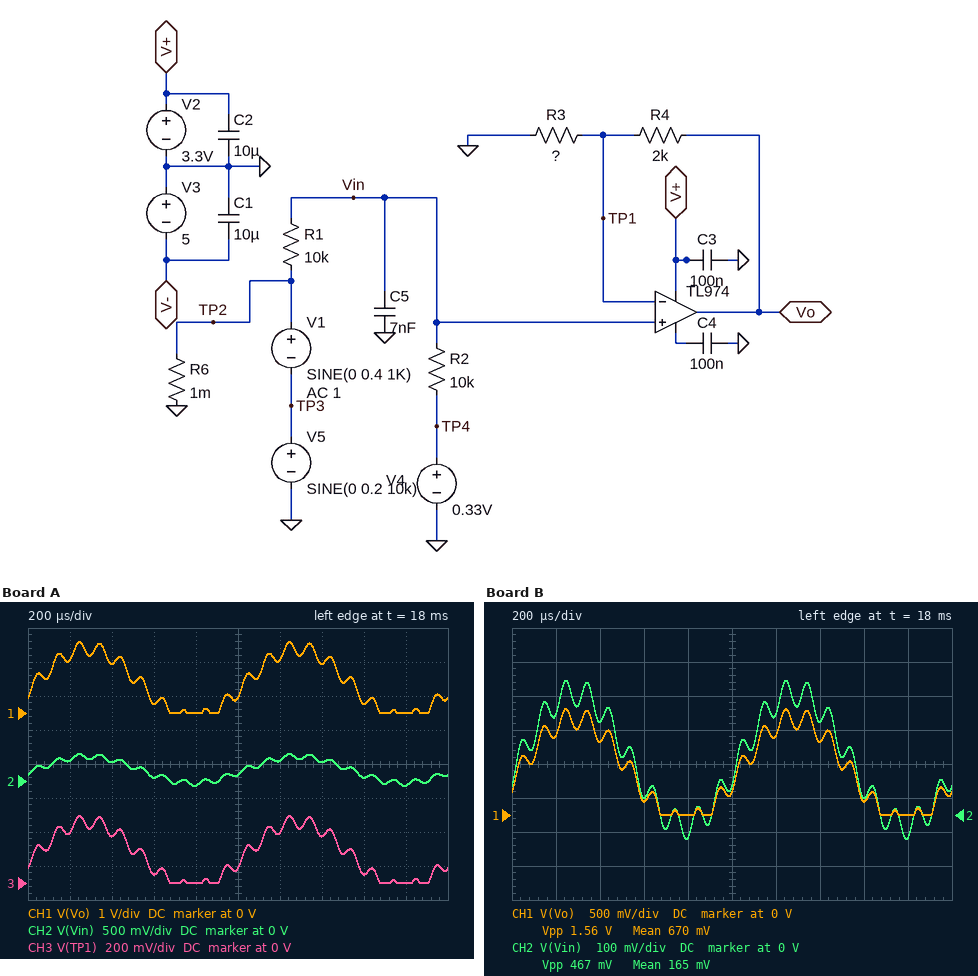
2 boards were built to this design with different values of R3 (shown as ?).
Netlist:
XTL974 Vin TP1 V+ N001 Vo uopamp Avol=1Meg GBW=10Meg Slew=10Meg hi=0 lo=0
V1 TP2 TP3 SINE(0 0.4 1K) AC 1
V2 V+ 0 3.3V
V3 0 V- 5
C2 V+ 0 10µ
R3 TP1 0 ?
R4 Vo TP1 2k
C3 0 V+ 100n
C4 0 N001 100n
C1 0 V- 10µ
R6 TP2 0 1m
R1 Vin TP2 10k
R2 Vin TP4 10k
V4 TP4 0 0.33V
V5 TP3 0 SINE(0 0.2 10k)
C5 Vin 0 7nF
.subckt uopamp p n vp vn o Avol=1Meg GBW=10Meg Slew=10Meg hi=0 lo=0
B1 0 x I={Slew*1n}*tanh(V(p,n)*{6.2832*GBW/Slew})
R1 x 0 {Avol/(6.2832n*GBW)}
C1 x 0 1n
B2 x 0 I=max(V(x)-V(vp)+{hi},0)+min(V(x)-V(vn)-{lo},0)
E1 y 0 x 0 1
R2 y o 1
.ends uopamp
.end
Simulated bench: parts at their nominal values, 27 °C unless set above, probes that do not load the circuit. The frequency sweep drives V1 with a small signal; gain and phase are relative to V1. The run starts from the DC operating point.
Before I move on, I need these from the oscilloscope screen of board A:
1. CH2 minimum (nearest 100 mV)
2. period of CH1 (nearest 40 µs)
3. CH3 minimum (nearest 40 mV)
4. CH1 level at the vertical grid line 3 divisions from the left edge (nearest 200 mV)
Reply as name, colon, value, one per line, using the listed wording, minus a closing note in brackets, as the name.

CH2 minimum: -100 mV
period of CH1: 1.00 ms
CH3 minimum: 0 V
CH1 level at the vertical grid line 3 divisions from the left edge: 200 mV
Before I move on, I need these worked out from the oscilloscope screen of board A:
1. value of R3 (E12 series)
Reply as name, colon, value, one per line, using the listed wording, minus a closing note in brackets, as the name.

value of R3: 470 Ω
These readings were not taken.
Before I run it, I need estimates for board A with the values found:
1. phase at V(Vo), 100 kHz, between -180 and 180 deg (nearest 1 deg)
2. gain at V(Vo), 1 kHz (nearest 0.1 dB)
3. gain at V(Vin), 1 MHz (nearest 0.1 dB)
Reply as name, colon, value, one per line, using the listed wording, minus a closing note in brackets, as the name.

phase at V(Vo), 100 kHz, between -180 and 180 deg: -90 deg
gain at V(Vo), 1 kHz: 8.2 dB
gain at V(Vin), 1 MHz: -52.9 dB
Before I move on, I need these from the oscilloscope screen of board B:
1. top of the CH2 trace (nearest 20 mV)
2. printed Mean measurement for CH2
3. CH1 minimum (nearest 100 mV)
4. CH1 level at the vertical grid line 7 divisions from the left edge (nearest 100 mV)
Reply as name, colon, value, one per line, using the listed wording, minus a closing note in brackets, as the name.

top of the CH2 trace: 400 mV
printed Mean measurement for CH2: 165 mV
CH1 minimum: 0 V
CH1 level at the vertical grid line 7 divisions from the left edge: 1.1 V
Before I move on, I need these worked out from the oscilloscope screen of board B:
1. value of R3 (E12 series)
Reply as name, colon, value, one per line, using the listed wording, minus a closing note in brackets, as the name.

value of R3: 680 Ω
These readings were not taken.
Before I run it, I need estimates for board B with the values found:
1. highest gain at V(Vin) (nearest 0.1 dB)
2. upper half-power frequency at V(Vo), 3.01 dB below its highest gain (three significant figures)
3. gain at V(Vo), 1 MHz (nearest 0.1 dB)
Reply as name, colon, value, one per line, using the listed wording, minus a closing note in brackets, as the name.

highest gain at V(Vin): -6.0 dB
upper half-power frequency at V(Vo), 3.01 dB below its highest gain: 4.55 kHz
gain at V(Vo), 1 MHz: -41.6 dB
